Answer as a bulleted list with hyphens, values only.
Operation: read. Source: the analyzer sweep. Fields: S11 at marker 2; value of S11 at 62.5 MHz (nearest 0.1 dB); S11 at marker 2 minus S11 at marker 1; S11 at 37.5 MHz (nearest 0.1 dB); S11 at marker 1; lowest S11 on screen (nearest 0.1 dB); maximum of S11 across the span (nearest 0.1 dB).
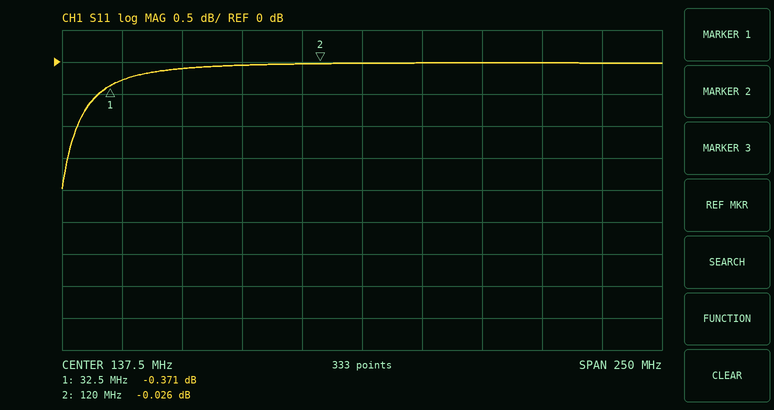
- -0.026 dB
- -0.1 dB
- 0.345 dB
- -0.3 dB
- -0.371 dB
- -2.0 dB
- 0.0 dB
